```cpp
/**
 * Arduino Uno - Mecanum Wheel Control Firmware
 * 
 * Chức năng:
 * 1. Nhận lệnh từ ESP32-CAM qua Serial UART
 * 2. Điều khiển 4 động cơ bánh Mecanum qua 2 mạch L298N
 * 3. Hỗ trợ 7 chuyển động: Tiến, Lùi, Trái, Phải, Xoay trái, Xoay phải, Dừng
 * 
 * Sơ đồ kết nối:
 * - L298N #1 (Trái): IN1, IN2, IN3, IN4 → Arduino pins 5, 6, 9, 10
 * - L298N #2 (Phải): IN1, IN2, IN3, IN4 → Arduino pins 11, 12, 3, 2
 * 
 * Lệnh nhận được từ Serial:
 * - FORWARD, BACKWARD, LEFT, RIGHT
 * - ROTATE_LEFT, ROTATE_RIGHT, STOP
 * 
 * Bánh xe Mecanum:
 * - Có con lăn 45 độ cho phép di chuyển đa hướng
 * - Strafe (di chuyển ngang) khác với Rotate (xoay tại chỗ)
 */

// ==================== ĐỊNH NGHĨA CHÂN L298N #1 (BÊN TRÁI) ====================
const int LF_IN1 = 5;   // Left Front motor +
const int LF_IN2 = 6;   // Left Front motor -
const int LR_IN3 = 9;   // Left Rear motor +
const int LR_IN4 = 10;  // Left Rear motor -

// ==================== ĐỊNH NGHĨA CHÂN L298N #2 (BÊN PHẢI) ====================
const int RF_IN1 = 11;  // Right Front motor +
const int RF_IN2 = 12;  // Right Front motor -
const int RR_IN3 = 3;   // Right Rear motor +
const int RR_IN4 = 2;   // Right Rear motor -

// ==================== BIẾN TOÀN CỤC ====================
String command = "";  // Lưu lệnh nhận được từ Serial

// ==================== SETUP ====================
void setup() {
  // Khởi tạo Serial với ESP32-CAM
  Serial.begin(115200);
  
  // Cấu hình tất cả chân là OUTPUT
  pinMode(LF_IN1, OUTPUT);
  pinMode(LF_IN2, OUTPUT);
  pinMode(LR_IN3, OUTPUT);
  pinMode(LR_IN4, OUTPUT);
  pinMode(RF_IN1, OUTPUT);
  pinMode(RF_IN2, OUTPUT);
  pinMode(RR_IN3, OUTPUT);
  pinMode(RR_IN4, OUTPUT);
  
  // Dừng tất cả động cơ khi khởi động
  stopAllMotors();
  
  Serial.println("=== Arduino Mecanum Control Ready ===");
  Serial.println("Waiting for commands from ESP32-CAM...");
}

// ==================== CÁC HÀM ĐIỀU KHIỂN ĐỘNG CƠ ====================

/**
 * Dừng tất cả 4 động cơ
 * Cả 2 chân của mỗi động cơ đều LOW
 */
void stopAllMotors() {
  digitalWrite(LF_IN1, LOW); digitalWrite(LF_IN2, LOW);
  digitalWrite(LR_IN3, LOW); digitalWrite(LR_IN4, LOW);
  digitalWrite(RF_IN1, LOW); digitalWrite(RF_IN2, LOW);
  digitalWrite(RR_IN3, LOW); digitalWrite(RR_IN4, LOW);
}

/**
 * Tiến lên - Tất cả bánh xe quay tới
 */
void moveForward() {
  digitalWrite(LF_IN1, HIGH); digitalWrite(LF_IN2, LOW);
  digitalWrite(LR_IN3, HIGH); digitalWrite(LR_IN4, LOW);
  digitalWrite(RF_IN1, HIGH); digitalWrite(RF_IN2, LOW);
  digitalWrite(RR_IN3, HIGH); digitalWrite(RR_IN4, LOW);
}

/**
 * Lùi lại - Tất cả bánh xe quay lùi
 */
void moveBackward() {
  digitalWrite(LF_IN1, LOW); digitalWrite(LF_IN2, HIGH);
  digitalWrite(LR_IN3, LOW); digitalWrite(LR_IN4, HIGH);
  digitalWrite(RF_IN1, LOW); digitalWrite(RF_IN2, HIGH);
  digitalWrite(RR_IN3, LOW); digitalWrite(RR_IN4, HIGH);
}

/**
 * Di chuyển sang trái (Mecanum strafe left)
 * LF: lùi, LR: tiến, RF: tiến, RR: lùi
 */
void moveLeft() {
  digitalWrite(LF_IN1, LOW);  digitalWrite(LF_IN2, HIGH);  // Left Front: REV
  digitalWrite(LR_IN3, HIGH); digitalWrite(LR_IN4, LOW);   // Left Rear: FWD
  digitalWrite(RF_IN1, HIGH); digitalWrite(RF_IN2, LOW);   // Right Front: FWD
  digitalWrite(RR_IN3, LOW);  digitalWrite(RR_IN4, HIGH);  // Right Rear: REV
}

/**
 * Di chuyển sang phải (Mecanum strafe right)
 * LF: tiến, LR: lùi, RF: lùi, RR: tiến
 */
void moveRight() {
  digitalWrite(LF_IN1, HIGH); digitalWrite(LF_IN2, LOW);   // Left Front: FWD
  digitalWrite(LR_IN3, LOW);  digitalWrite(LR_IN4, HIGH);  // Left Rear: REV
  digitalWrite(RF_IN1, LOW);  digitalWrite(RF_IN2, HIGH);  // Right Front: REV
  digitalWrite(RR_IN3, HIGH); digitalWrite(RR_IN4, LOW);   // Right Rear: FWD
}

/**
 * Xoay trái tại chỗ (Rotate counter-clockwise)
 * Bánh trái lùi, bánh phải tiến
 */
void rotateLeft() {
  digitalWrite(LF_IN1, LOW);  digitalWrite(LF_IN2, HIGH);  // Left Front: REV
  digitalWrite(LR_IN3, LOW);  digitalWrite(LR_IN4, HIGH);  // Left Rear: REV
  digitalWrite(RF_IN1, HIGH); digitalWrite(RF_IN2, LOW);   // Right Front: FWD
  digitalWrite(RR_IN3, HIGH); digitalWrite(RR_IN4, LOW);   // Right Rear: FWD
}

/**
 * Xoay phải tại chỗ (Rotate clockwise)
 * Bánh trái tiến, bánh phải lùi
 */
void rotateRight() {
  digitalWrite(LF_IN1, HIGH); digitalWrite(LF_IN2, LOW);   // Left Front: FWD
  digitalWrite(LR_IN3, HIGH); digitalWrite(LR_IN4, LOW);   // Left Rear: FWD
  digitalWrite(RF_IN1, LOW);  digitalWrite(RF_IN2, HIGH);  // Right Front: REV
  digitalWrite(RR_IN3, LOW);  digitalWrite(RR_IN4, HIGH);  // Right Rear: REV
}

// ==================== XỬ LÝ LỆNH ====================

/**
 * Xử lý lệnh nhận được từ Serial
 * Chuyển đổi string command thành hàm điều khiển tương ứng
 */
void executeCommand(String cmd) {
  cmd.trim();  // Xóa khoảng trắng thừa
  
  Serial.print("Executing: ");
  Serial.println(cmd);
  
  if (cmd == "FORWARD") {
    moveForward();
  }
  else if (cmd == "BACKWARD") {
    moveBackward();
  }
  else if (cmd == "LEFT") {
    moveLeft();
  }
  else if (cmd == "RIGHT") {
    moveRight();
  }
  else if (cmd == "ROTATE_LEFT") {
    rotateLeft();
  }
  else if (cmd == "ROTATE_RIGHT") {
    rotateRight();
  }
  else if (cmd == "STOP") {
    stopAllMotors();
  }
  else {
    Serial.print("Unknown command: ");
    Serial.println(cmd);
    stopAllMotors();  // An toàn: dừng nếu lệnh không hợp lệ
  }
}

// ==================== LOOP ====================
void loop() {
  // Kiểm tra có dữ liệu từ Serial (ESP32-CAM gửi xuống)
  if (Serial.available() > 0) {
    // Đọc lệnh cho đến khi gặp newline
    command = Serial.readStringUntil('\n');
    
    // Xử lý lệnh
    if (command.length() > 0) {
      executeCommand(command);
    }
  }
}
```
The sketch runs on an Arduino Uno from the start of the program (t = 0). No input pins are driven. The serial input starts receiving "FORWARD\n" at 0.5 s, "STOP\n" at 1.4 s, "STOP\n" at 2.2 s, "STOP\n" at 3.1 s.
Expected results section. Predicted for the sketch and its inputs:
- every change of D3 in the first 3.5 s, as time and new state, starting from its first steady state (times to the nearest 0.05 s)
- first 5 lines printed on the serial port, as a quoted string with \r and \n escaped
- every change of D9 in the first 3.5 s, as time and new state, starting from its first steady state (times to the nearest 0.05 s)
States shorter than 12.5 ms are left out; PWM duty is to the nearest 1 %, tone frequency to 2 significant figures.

0 s low; 0.5 s high; 1.4 s low
"=== Arduino Mecanum Control Ready ===\r\nWaiting for commands from ESP32-CAM...\r\nExecuting: FORWARD\r\nExecuting: STOP\r\nExecuting: STOP\r\n"
0 s low; 0.5 s high; 1.4 s low
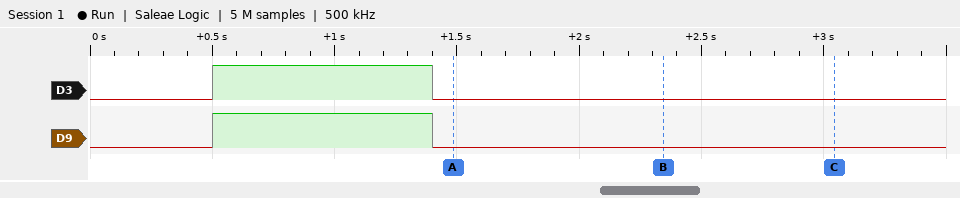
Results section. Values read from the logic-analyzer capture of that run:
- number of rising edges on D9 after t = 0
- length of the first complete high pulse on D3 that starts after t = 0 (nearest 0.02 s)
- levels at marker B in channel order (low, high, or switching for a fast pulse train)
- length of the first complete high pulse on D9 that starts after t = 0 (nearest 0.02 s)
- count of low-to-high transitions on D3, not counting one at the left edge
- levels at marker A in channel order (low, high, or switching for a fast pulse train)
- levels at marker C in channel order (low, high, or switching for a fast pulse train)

1
0.90 s
D3 low, D9 low
0.90 s
1
D3 low, D9 low
D3 low, D9 low
